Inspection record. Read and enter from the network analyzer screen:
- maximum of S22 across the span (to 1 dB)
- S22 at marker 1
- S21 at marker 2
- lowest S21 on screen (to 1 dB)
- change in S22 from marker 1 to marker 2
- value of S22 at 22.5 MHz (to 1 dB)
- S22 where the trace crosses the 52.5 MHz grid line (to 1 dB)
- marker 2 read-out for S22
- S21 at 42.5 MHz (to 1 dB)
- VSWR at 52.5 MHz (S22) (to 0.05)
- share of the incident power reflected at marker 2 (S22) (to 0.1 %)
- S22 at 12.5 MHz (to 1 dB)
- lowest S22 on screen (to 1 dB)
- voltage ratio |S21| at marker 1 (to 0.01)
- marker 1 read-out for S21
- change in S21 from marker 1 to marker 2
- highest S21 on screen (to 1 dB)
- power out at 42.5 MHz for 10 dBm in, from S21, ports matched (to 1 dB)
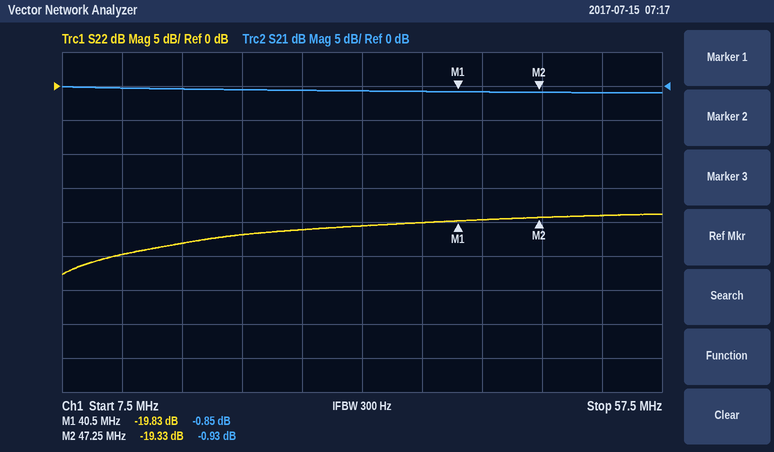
-19 dB
-19.83 dB
-0.93 dB
-1 dB
0.50 dB
-22 dB
-19 dB
-19.33 dB
-1 dB
1.25
1.2 %
-25 dB
-28 dB
0.91
-0.85 dB
-0.08 dB
0 dB
9 dBm
